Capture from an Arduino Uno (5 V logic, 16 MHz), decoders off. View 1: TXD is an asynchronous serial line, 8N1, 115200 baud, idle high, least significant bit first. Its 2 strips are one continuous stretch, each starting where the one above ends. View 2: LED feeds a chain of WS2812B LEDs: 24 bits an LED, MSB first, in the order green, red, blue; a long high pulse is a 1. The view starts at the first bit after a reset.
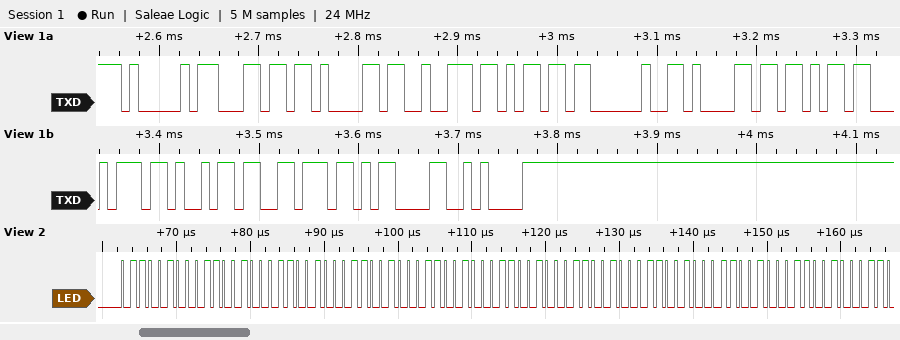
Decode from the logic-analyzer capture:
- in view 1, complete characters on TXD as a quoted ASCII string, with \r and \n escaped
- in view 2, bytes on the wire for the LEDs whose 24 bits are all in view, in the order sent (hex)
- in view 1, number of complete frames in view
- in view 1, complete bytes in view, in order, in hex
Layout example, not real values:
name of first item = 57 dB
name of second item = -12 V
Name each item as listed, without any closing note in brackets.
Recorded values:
in view 1, complete characters on TXD as a quoted ASCII string, with \r and \n escaped = "Alarm aktiv\r\n"
in view 2, bytes on the wire for the LEDs whose 24 bits are all in view, in the order sent = 64 64 64 64 64 64 64 64 64
in view 1, number of complete frames in view = 13
in view 1, complete bytes in view, in order, in hex = 41 6C 61 72 6D 20 61 6B 74 69 76 0D 0A
